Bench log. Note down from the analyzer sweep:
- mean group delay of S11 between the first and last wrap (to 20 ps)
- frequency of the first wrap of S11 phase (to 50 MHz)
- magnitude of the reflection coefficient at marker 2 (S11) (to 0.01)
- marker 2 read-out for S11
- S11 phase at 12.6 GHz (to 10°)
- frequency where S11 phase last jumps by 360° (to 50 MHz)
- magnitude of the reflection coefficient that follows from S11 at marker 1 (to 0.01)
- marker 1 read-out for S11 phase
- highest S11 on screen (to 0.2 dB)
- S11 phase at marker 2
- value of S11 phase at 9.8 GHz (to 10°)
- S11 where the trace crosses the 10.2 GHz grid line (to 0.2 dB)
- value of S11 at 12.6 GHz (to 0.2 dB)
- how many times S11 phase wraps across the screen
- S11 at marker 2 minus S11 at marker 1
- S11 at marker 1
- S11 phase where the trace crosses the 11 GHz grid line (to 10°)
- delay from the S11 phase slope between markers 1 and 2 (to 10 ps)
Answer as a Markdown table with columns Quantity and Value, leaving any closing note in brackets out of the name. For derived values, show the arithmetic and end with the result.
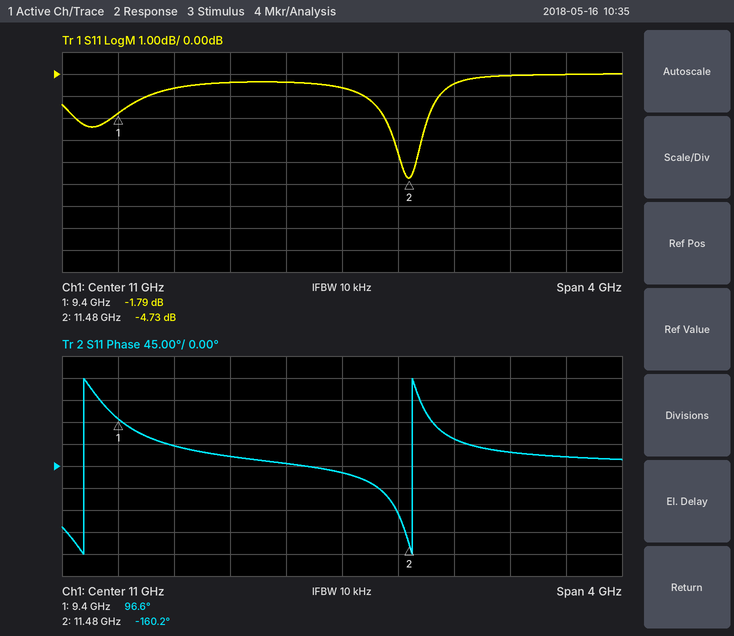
| Quantity | Value |
|---|---|
| mean group delay of S11 between the first and last wrap | 1 cycle / (11.50 GHz − 9.15 GHz) ≈ 426 ps, so 420 ps to the nearest 20 ps |
| frequency of the first wrap of S11 phase | 9.15 GHz |
| magnitude of the reflection coefficient at marker 2 (S11) | 10^(-4.73/20) ≈ 0.58 |
| marker 2 read-out for S11 | -4.73 dB |
| S11 phase at 12.6 GHz | 20° |
| frequency where S11 phase last jumps by 360° | 11.50 GHz |
| magnitude of the reflection coefficient that follows from S11 at marker 1 | 10^(-1.79/20) ≈ 0.81 |
| marker 1 read-out for S11 phase | 96.6° |
| highest S11 on screen | 0.0 dB |
| S11 phase at marker 2 | -160.2° |
| value of S11 phase at 9.8 GHz | 40° |
| S11 where the trace crosses the 10.2 GHz grid line | -0.4 dB |
| value of S11 at 12.6 GHz | 0.0 dB |
| how many times S11 phase wraps across the screen | 2 |
| S11 at marker 2 minus S11 at marker 1 | -4.73 − (-1.79) = -2.94 dB |
| S11 at marker 1 | -1.79 dB |
| S11 phase where the trace crosses the 11 GHz grid line | -10° |
| delay from the S11 phase slope between markers 1 and 2 | −(-160.2° − (96.6°))/(360° × 2.08 GHz) ≈ 343 ps, so 340 ps to the nearest 10 ps |
